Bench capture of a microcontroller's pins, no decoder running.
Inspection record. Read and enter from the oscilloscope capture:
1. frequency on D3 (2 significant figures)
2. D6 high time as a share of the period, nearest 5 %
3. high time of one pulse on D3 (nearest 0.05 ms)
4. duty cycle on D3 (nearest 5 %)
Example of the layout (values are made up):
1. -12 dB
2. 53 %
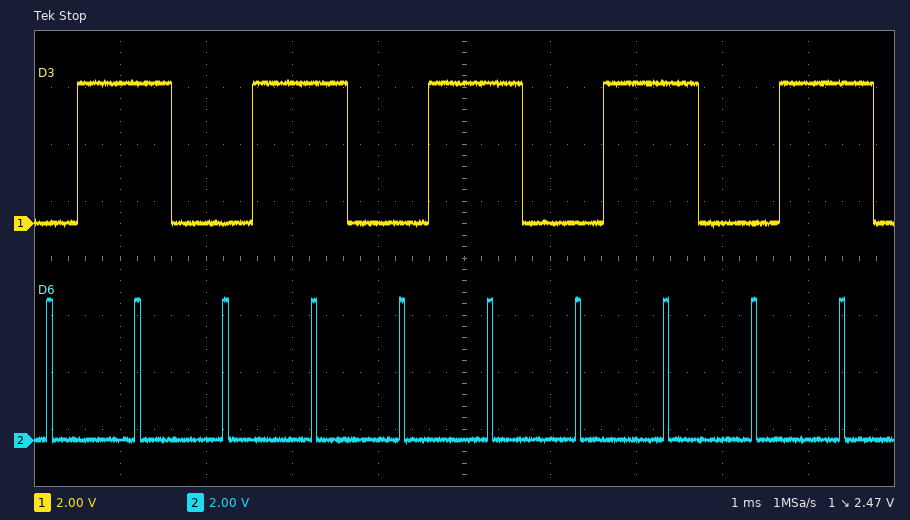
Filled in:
1. 490 Hz
2. 5 %
3. 1.10 ms
4. 55 %
